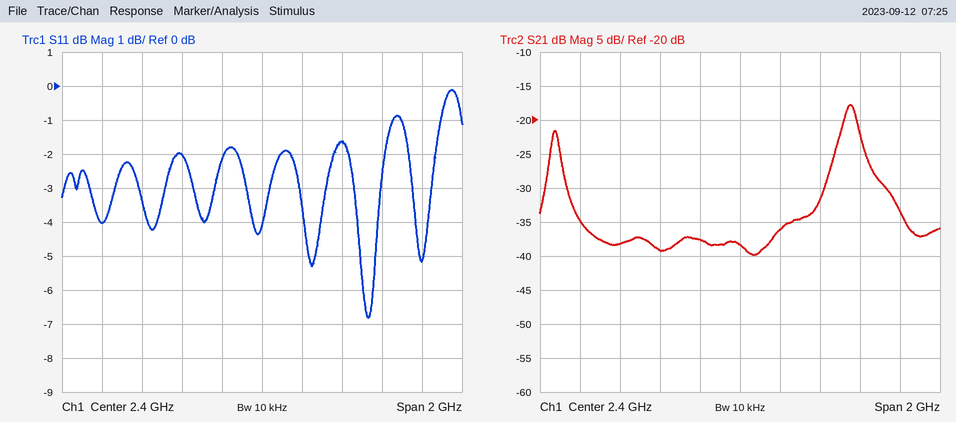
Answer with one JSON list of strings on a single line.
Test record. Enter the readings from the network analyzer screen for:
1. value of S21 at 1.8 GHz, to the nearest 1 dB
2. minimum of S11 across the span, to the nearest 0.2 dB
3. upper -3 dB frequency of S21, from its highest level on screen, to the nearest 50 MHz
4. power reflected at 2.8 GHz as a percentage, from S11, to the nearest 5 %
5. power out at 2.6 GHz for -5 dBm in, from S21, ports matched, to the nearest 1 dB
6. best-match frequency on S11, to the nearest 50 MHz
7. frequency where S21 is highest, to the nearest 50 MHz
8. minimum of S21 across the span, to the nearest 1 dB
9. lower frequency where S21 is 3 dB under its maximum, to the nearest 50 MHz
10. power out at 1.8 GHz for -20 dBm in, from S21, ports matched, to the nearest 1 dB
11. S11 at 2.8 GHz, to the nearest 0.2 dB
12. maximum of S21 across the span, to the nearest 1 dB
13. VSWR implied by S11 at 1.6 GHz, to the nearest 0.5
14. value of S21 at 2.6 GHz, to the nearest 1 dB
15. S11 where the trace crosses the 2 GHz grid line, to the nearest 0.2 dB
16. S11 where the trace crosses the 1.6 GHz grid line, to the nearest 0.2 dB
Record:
["-38 dB", "-6.8 dB", "3.00 GHz", "70 %", "-41 dBm", "2.95 GHz", "2.95 GHz", "-40 dB", "2.90 GHz", "-58 dBm", "-1.6 dB", "-18 dB", "4.5", "-36 dB", "-2.0 dB", "-4.0 dB"]
